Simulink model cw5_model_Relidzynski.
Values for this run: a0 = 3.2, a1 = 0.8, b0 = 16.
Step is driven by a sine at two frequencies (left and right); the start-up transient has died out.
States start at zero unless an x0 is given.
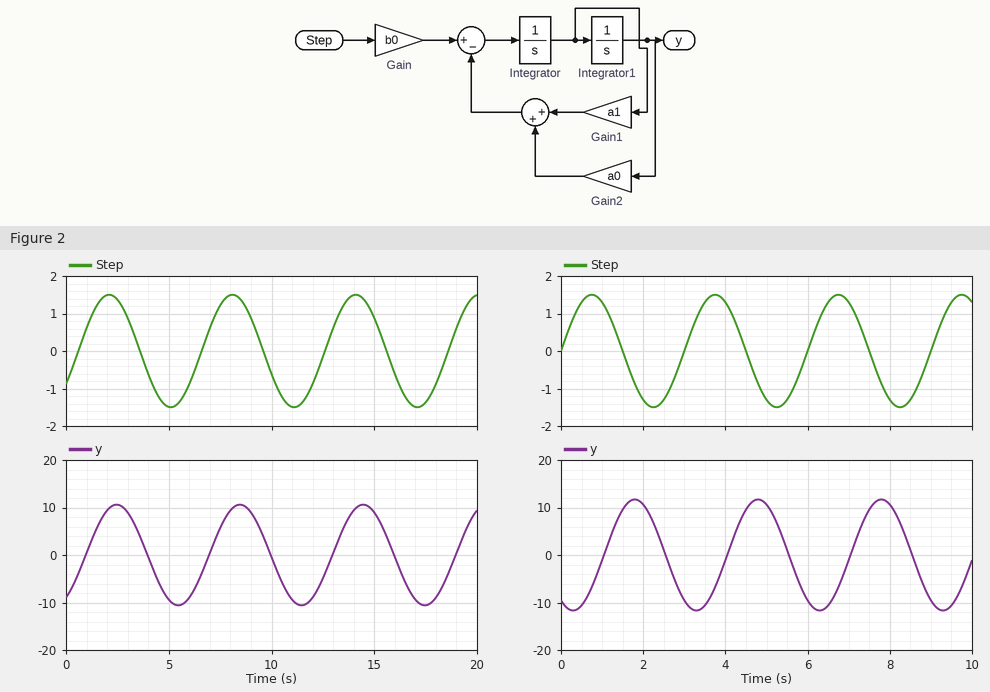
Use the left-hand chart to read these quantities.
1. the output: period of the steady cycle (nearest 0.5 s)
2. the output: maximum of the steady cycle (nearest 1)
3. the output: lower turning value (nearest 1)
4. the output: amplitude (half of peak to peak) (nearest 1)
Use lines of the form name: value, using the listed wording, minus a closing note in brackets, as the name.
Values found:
the output: period of the steady cycle: 6.0 s
the output: maximum of the steady cycle: 11
the output: lower turning value: -11
the output: amplitude (half of peak to peak): 11
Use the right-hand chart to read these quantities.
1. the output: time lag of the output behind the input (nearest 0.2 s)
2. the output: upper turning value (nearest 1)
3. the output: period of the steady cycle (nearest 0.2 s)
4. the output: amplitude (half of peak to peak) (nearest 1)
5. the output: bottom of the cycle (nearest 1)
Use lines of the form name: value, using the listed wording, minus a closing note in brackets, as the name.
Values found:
the output: time lag of the output behind the input: 1.0 s
the output: upper turning value: 12
the output: period of the steady cycle: 3.0 s
the output: amplitude (half of peak to peak): 12
the output: bottom of the cycle: -12
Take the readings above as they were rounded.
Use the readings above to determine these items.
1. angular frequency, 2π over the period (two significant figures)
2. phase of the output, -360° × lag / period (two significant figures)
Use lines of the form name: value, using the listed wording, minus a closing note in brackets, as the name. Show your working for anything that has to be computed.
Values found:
angular frequency, 2π over the period: 2π / 3 = 2.1 rad/s
phase of the output, -360° × lag / period: -360 × 1 / 3 = -120°
